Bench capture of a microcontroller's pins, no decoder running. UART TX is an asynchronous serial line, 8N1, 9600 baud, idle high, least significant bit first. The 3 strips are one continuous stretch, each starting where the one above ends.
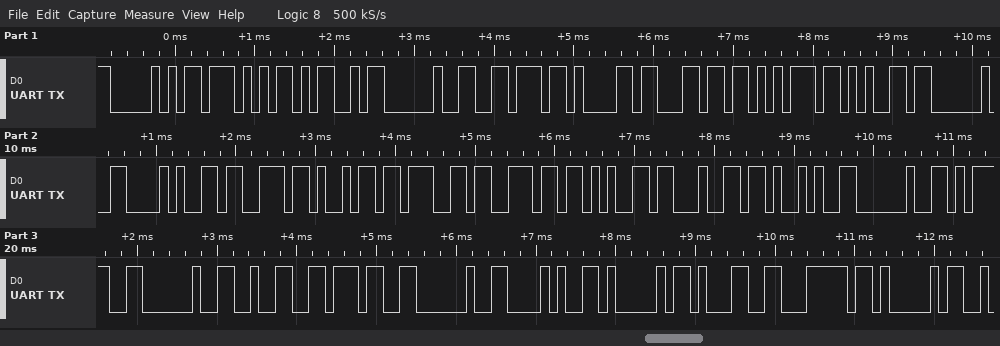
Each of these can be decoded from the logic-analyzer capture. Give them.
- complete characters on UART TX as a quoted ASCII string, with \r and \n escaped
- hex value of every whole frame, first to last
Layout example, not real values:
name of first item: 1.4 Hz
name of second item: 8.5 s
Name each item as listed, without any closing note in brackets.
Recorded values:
complete characters on UART TX as a quoted ASCII string, with \r and \n escaped: "PWM value (signed) = 27 (A1|A"
hex value of every whole frame, first to last: 50 57 4D 20 76 61 6C 75 65 20 28 73 69 67 6E 65 64 29 20 3D 20 32 37 20 28 41 31 7C 41
